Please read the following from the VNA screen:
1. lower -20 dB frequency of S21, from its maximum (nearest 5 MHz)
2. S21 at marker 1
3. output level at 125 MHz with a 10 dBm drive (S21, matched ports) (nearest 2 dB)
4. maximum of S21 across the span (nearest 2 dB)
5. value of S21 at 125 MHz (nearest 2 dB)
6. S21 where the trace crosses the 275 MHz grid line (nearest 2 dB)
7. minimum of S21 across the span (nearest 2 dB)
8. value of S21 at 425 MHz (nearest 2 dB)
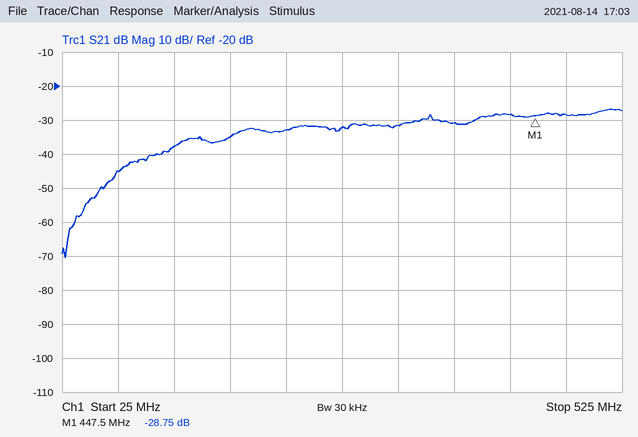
70 MHz
-28.75 dB
-28 dBm
-26 dB
-38 dB
-32 dB
-70 dB
-28 dB
